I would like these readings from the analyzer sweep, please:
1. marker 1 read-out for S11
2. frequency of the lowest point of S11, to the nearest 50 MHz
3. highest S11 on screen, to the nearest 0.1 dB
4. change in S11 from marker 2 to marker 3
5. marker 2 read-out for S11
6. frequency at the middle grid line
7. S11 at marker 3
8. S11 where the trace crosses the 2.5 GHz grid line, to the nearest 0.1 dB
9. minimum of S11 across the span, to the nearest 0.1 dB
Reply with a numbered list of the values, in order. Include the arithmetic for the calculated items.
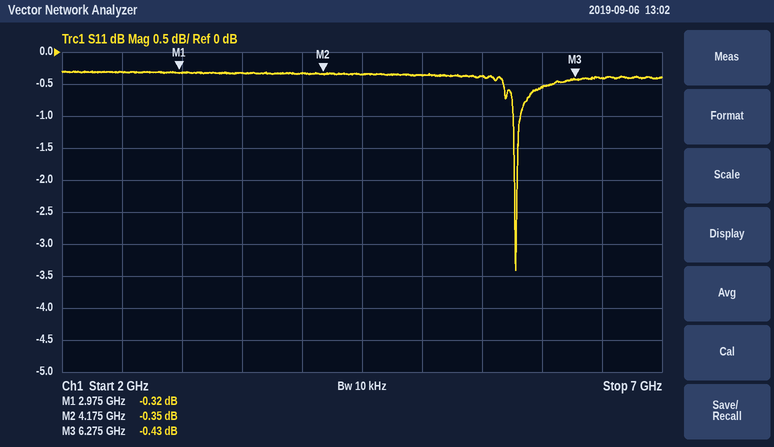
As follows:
1. -0.32 dB
2. 5.80 GHz
3. -0.3 dB
4. -0.43 − (-0.35) = -0.08 dB
5. -0.35 dB
6. 4.5 GHz
7. -0.43 dB
8. -0.3 dB
9. -3.4 dB
